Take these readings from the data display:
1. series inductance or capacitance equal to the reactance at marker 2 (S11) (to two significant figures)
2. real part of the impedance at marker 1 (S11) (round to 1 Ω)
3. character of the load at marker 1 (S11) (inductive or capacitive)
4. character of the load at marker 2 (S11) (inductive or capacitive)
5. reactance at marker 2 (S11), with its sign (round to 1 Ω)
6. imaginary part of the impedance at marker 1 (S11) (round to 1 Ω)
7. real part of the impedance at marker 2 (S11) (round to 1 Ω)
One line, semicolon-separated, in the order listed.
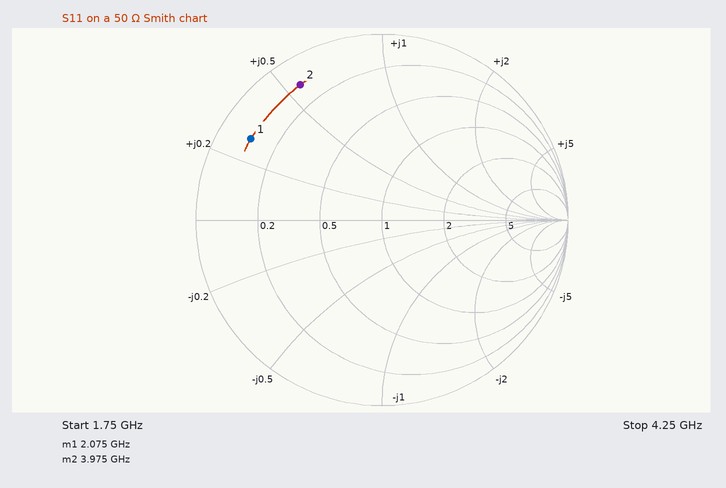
1.1 nH; 5 Ω; inductive; inductive; +28 Ω; +14 Ω; 5 Ω
